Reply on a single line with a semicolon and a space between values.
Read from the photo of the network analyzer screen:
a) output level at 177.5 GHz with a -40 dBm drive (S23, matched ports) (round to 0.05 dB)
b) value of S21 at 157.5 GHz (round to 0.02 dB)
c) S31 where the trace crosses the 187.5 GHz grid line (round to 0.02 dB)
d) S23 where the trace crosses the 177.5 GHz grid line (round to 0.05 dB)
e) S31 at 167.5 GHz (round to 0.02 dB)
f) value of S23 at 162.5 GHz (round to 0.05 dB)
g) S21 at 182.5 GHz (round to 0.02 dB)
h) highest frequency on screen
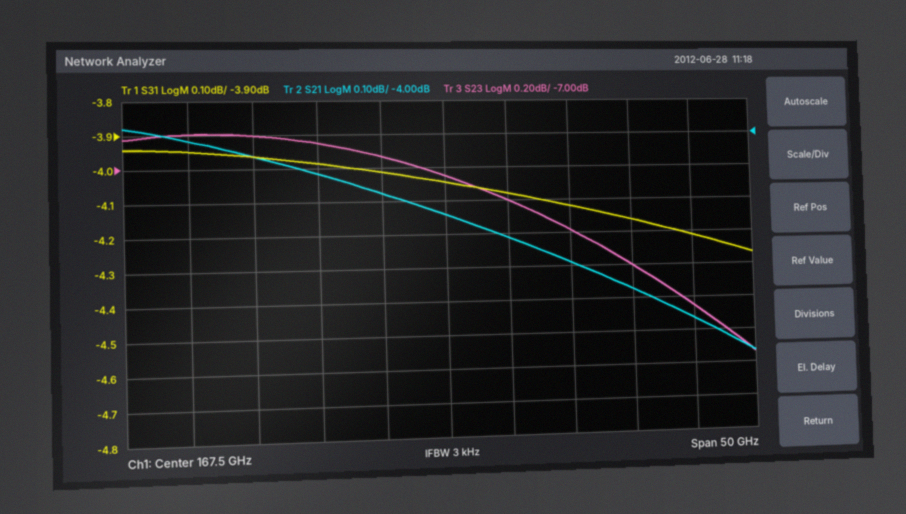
-47.40 dBm; -4.12 dB; -4.22 dB; -7.40 dB; -4.04 dB; -6.95 dB; -4.48 dB; 192.5 GHz
